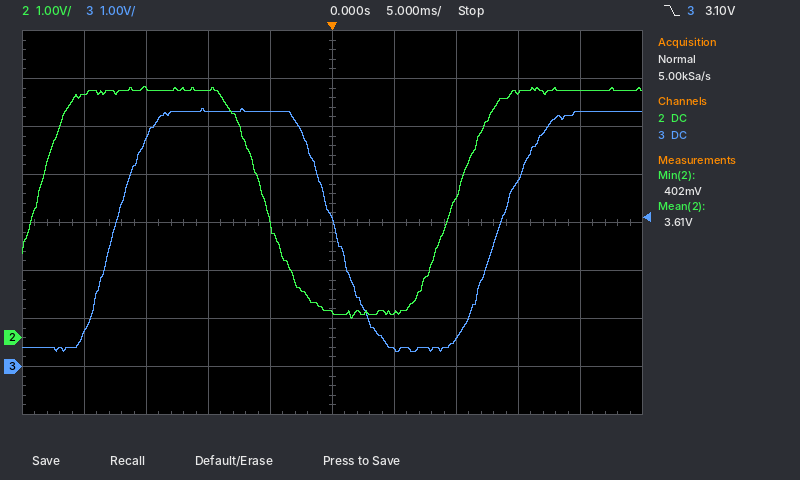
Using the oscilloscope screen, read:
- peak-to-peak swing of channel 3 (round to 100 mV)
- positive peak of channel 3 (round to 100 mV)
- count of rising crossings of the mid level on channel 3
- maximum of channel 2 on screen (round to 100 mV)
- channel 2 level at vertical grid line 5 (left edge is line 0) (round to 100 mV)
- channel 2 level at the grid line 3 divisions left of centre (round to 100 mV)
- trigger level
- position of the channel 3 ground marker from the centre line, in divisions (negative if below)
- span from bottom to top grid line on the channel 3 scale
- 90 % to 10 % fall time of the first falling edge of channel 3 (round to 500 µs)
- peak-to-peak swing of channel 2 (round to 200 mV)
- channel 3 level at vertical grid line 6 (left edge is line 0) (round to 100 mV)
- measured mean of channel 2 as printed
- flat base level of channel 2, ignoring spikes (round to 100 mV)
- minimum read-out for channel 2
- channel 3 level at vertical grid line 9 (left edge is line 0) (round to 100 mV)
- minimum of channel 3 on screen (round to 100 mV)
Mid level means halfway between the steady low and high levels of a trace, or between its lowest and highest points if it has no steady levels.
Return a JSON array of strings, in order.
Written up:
["5.1 V", "5.4 V", "2", "5.2 V", "500 mV", "5.2 V", "3.10 V", "-3.0 div", "8 V", "5.5 ms", "4.8 V", "400 mV", "3.61 V", "500 mV", "402 mV", "5.3 V", "300 mV"]
